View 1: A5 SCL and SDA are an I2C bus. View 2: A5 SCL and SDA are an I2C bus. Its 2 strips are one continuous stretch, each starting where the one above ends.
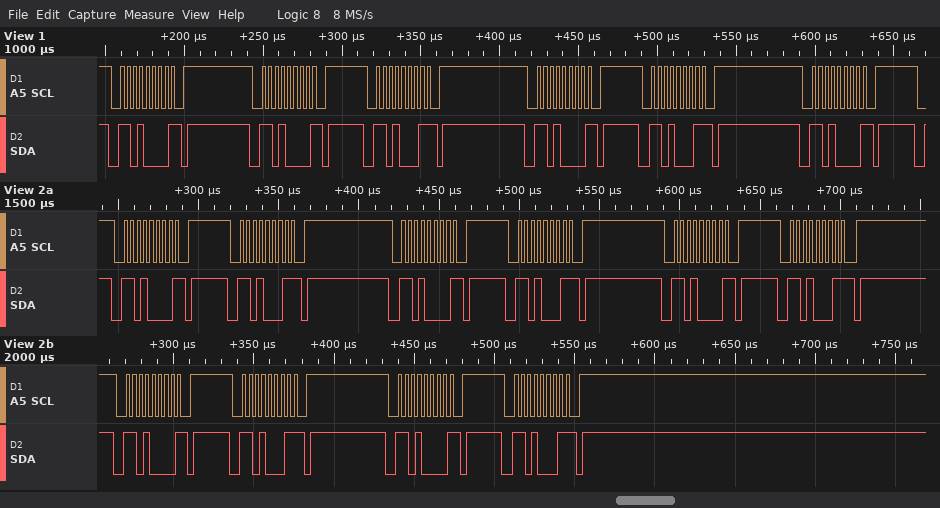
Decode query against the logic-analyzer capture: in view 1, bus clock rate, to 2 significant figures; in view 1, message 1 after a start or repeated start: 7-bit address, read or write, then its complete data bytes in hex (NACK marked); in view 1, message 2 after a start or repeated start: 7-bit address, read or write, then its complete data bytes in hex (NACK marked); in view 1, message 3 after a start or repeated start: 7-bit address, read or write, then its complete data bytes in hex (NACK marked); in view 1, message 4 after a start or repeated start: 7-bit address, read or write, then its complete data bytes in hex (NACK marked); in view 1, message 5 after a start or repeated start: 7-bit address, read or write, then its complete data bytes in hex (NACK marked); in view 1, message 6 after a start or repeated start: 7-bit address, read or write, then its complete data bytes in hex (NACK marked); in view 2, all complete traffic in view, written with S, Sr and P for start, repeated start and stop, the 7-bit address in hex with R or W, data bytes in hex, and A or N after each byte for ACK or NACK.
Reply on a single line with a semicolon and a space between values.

250 kHz; 0x68 write NACK; 0x68 write NACK; 0x68 read NACK; 0x68 write NACK; 0x68 read NACK; 0x68 write NACK; S 68W N P S 68R N P S 68W N P S 68R N P S 68W N P S 68R N P S 68W N P S 68R N P S 68W N P S 68R N P
